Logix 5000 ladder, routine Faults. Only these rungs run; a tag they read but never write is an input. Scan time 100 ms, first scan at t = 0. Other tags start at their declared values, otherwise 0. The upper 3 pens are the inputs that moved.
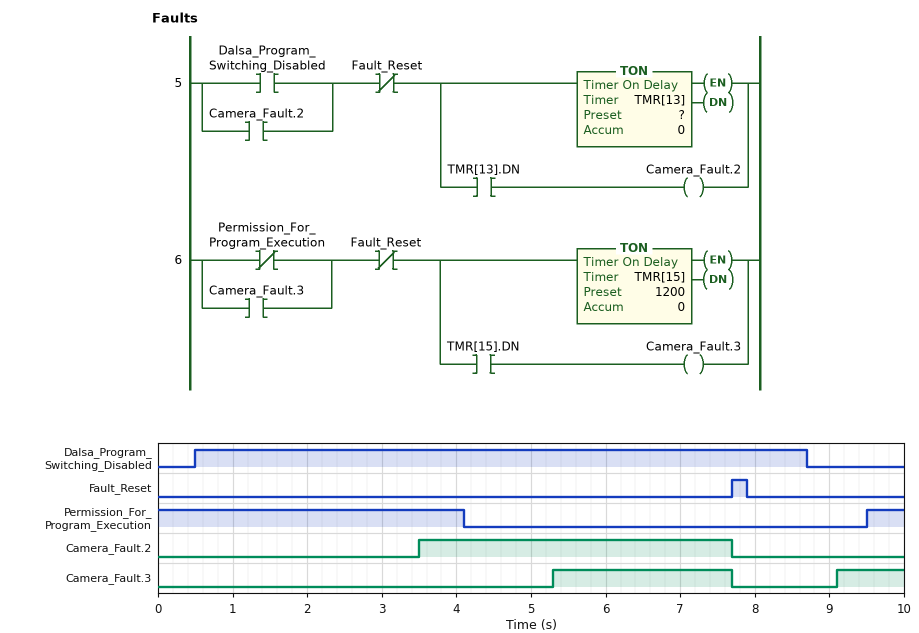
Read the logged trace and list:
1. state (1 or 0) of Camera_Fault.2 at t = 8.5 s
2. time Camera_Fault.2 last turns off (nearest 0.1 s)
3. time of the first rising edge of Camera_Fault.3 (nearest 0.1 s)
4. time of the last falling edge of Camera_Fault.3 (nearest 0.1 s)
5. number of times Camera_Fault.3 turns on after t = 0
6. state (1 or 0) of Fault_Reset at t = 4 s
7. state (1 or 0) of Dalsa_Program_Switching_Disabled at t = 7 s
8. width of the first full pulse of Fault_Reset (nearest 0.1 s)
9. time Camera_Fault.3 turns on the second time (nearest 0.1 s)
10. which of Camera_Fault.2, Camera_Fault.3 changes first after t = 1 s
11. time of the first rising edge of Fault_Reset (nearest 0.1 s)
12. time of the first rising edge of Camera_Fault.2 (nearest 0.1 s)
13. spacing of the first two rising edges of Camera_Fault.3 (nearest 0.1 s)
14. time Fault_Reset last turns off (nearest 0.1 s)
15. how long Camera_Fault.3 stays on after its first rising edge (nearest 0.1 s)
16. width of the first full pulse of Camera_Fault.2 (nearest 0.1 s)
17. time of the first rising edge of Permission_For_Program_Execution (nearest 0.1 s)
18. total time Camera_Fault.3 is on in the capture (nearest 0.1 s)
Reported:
0
7.7 s
5.3 s
7.7 s
2
0
1
0.2 s
9.1 s
Camera_Fault.2
7.7 s
3.5 s
3.8 s
7.9 s
2.4 s
4.2 s
9.5 s
3.3 s
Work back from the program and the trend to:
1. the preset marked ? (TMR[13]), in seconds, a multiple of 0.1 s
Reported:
3.0 s
